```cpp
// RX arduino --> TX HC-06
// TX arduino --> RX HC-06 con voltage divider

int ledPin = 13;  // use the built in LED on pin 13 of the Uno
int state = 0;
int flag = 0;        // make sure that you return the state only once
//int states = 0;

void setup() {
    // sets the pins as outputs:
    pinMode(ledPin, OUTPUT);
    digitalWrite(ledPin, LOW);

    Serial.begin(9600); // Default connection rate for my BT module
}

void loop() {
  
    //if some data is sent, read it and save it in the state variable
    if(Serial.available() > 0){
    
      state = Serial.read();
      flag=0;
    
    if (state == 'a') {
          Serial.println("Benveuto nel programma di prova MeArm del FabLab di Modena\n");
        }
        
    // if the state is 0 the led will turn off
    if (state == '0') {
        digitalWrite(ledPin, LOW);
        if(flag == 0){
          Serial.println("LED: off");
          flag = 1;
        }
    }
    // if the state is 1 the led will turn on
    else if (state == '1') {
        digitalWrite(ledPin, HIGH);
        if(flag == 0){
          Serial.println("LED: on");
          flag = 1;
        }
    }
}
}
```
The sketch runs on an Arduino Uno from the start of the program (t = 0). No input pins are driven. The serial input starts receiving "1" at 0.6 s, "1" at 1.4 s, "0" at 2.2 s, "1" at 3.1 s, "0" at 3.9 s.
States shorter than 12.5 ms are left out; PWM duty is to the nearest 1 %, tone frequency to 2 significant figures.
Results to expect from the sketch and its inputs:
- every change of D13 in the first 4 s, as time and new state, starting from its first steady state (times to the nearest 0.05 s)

0 s low; 0.6 s high; 2.2 s low; 3.1 s high; 3.9 s low
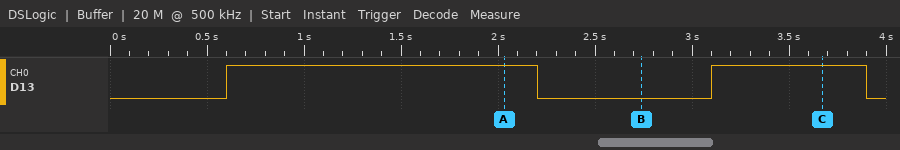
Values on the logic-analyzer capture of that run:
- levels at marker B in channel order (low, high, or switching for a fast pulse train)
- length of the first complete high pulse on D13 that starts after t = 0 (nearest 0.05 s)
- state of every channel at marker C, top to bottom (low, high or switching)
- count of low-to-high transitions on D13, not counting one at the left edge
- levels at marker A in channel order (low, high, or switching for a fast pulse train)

D13 low
1.60 s
D13 high
2
D13 high
